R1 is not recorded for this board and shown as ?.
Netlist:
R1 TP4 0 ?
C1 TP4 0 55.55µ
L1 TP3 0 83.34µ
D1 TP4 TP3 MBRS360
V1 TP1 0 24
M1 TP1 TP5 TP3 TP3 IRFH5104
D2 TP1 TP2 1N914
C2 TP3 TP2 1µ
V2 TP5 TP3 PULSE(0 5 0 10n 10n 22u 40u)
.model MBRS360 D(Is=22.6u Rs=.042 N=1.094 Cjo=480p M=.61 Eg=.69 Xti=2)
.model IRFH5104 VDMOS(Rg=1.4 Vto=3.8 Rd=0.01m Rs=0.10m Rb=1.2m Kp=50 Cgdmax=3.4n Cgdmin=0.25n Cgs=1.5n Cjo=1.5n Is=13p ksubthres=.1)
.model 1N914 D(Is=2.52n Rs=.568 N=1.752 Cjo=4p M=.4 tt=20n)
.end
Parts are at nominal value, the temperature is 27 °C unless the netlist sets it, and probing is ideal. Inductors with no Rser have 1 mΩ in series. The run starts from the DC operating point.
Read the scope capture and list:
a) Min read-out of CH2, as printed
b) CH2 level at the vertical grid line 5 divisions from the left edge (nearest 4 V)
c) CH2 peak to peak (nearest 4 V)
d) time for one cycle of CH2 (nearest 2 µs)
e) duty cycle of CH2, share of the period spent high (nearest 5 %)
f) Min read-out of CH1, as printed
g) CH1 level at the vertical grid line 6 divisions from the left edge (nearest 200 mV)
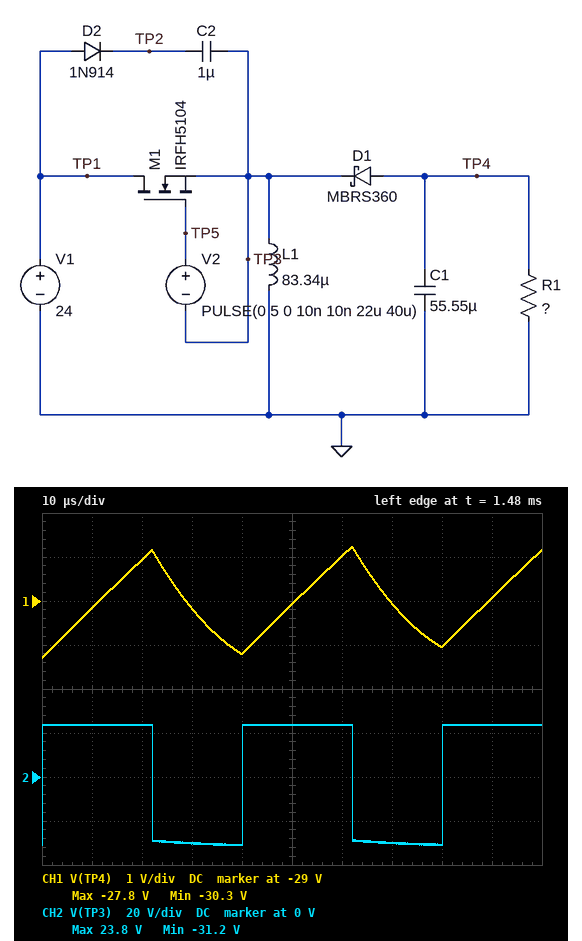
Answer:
-31.2 V
24 V
56 V
40 µs
55 %
-30.3 V
-28.0 V
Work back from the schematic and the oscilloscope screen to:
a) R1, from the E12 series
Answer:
4.7 Ω
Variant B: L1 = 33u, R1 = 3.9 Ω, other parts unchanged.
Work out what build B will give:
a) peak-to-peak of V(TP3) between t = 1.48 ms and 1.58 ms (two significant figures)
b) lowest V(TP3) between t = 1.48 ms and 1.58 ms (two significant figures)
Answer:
54 V
-30 V
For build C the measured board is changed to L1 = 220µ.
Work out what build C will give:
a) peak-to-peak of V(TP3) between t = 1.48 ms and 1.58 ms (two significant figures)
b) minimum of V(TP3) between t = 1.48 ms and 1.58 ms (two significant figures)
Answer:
53 V
-30 V
